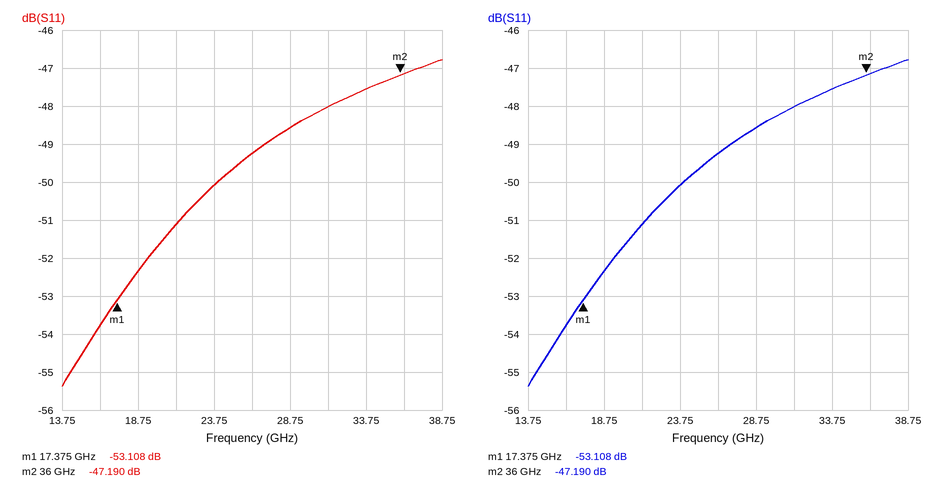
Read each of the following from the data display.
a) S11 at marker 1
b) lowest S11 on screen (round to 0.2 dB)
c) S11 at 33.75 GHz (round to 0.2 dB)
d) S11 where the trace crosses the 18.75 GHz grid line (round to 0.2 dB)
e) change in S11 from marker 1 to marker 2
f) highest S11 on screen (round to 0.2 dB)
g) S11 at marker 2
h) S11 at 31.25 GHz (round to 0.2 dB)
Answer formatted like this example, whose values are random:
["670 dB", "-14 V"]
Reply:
["-53.108 dB", "-55.4 dB", "-47.6 dB", "-52.4 dB", "5.918 dB", "-46.8 dB", "-47.190 dB", "-48.0 dB"]
